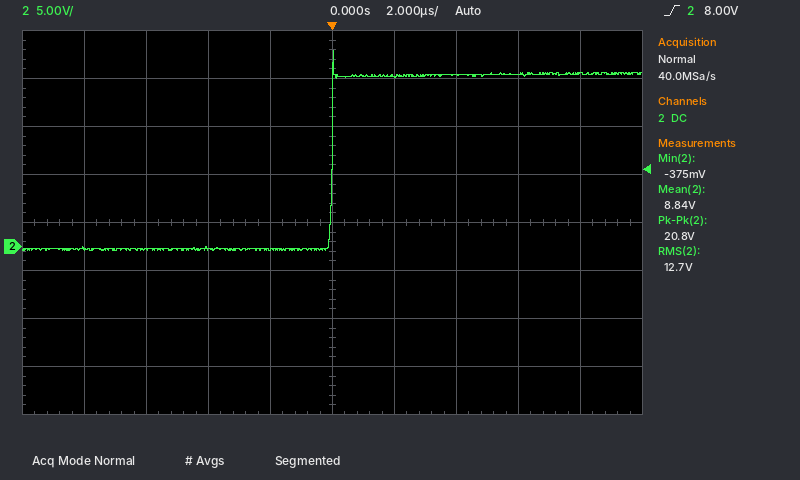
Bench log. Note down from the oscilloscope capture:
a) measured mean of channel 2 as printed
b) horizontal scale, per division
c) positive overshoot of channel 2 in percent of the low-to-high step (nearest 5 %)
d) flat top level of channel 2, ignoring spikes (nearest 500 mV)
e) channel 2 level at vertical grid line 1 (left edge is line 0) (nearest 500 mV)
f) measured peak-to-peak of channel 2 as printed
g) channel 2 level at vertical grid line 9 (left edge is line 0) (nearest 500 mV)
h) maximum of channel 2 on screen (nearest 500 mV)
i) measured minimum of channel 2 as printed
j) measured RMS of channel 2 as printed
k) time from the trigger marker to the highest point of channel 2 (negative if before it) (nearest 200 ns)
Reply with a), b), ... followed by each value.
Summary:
a) 8.84 V
b) 2 µs
c) 15 %
d) 18.0 V
e) 0.0 V
f) 20.8 V
g) 18.0 V
h) 20.5 V
i) -375 mV
j) 12.7 V
k) 0.0 µs
